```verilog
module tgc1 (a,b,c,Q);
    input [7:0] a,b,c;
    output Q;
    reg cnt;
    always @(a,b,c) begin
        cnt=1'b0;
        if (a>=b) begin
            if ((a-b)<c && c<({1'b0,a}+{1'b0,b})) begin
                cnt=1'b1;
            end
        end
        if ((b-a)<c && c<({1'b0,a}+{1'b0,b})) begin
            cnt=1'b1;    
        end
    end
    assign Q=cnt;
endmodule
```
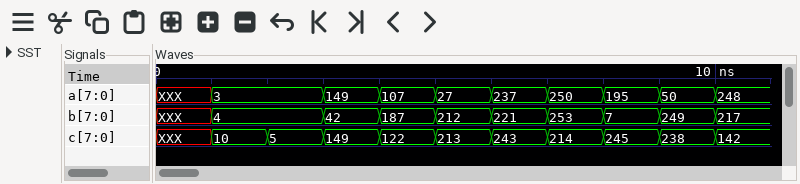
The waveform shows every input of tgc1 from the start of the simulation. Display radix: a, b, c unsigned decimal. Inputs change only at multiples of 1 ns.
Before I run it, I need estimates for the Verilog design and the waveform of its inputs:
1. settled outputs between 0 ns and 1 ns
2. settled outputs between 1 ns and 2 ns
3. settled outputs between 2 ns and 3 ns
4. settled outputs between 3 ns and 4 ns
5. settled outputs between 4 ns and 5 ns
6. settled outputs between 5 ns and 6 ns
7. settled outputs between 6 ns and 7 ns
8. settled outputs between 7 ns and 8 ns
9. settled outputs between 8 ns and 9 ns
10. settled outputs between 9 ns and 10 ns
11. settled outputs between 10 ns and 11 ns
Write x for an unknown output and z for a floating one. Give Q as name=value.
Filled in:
Q=x
Q=0
Q=1
Q=1
Q=1
Q=1
Q=1
Q=1
Q=0
Q=1
Q=1
